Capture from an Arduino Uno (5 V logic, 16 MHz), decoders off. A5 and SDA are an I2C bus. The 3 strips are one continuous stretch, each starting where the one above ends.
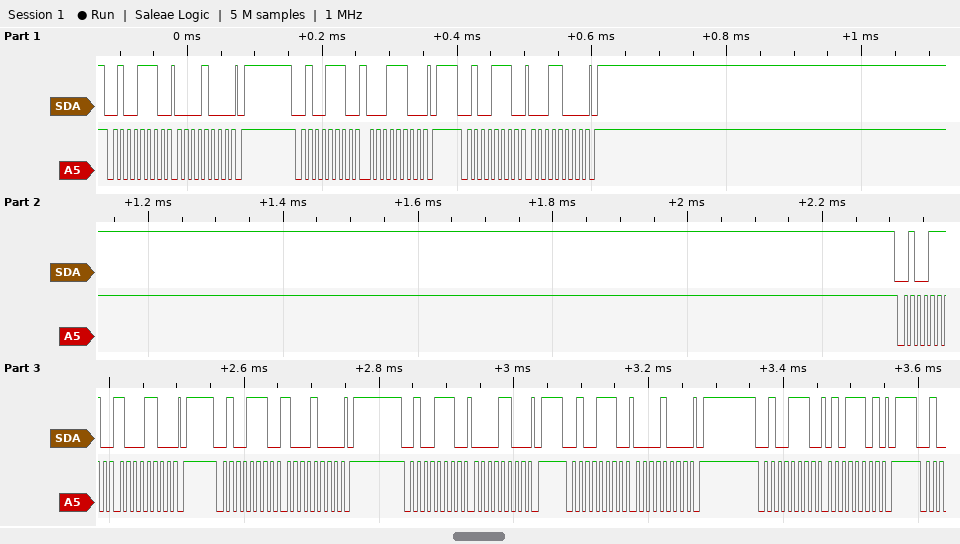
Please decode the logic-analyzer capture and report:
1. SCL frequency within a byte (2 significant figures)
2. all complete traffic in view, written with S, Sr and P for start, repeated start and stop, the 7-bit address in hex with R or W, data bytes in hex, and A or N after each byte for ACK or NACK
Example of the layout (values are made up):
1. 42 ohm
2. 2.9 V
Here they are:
1. 100 kHz
2. S 27W A 08 A P S 27W A 1C A P S 27W A 18 A P S 27W A 8C A P S 27W A 88 A P S 27W A 0C A P S 27W A 08 A P S 27W A 5D A P
